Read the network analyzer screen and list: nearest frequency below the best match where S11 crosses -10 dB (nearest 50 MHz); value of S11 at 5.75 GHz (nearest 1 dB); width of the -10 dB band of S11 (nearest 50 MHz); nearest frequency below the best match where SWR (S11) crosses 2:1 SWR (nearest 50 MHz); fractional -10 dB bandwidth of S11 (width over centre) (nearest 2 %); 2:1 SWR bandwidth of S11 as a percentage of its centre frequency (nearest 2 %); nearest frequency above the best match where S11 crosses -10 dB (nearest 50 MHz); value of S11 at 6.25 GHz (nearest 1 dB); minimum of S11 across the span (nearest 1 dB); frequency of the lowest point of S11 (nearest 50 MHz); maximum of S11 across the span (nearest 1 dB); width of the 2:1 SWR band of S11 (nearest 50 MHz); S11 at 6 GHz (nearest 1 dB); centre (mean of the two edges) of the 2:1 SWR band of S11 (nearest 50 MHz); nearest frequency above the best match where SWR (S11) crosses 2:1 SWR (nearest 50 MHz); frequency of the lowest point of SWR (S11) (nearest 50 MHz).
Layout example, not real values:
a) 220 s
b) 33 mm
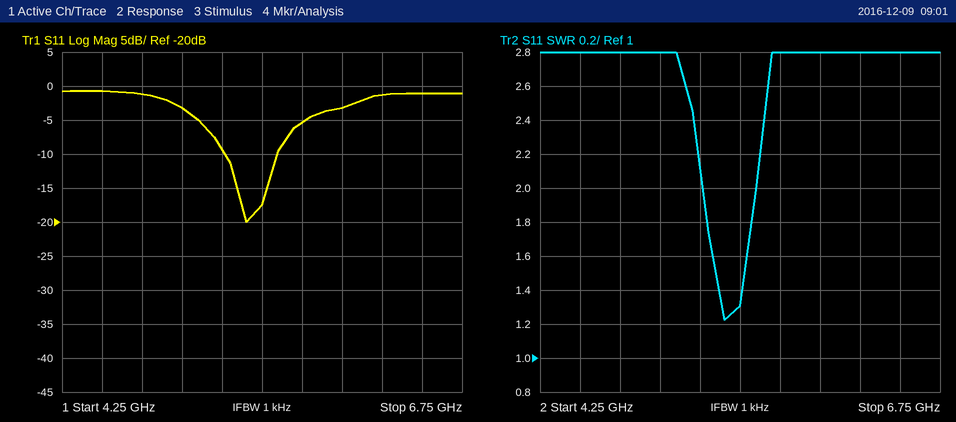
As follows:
a) 5.25 GHz
b) -5 dB
c) 350 MHz
d) 5.25 GHz
e) 6 %
f) 6 %
g) 5.60 GHz
h) -1 dB
i) -20 dB
j) 5.40 GHz
k) -1 dB
l) 350 MHz
m) -3 dB
n) 5.45 GHz
o) 5.60 GHz
p) 5.40 GHz
